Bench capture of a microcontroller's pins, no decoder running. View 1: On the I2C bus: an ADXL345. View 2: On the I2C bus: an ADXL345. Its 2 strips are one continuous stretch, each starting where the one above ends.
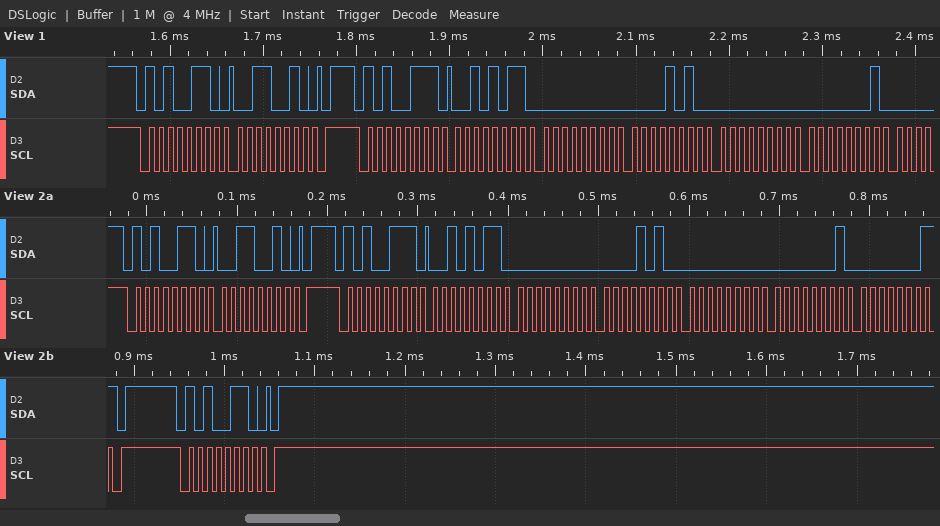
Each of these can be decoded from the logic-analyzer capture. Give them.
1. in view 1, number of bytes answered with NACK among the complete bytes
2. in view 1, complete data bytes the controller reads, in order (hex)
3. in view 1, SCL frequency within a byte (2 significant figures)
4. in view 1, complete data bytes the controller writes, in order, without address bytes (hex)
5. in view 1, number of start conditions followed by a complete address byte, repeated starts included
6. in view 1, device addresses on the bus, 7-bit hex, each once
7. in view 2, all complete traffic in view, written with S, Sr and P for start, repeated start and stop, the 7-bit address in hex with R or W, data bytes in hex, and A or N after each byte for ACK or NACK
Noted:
0
2B 00 0A 00 01
100 kHz
32
2
0x53
S 53W A 32 A P S 53R A 2B A 00 A 0A A 00 A 01 A 01 N P S 53W A P
